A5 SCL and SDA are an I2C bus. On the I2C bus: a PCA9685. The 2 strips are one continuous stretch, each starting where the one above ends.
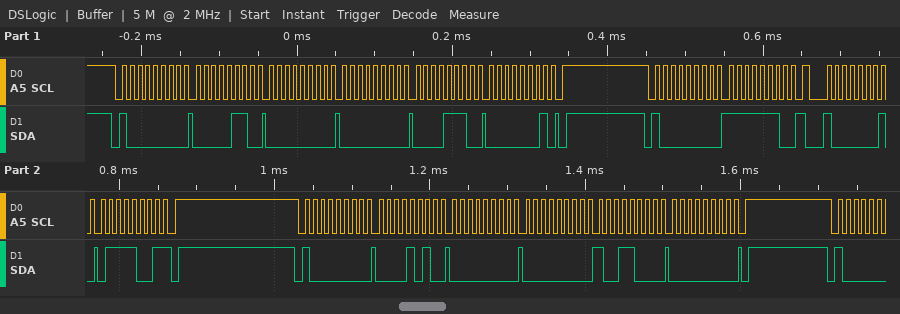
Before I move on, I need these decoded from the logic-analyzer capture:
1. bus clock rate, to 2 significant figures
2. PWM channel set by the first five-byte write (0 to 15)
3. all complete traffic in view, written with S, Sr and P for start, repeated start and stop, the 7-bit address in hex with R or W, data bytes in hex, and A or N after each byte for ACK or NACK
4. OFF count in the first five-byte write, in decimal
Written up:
100 kHz
0
S 40W A 06 A 00 A 00 A 0E A 01 A P S 40W A FE A Sr 40R A 79 N P S 40W A 0A A 00 A 00 A 98 A 00 A P
270
